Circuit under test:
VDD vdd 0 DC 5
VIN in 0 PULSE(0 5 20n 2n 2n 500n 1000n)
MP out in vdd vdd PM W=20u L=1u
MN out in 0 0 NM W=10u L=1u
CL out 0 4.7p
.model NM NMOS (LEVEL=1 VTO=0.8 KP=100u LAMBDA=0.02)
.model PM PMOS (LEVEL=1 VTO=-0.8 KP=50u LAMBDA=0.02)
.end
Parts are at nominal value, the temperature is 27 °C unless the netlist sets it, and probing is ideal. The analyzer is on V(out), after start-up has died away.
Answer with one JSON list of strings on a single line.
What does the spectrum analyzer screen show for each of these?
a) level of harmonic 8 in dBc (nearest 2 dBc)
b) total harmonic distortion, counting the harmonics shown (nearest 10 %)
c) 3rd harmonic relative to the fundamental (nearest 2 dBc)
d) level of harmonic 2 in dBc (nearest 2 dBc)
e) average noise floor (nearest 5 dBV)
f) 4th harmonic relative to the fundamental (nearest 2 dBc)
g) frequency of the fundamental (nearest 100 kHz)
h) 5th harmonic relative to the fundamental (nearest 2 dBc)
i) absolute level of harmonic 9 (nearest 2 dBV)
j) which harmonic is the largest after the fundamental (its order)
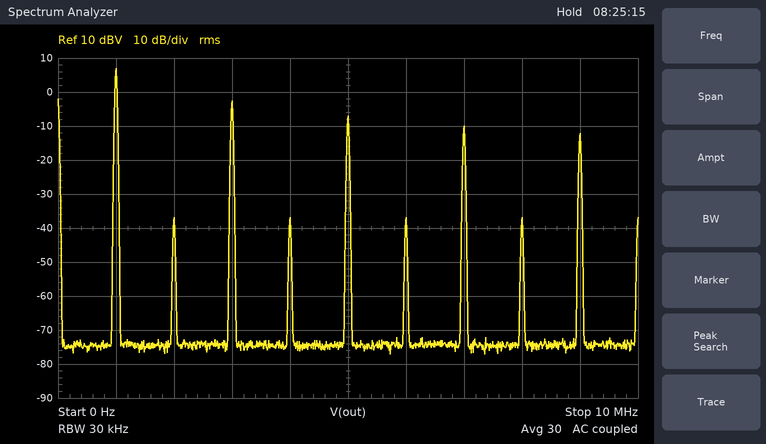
["-44 dBc", "40 %", "-10 dBc", "-44 dBc", "-75 dBV", "-44 dBc", "1.0 MHz", "-14 dBc", "-12 dBV", "3"]
